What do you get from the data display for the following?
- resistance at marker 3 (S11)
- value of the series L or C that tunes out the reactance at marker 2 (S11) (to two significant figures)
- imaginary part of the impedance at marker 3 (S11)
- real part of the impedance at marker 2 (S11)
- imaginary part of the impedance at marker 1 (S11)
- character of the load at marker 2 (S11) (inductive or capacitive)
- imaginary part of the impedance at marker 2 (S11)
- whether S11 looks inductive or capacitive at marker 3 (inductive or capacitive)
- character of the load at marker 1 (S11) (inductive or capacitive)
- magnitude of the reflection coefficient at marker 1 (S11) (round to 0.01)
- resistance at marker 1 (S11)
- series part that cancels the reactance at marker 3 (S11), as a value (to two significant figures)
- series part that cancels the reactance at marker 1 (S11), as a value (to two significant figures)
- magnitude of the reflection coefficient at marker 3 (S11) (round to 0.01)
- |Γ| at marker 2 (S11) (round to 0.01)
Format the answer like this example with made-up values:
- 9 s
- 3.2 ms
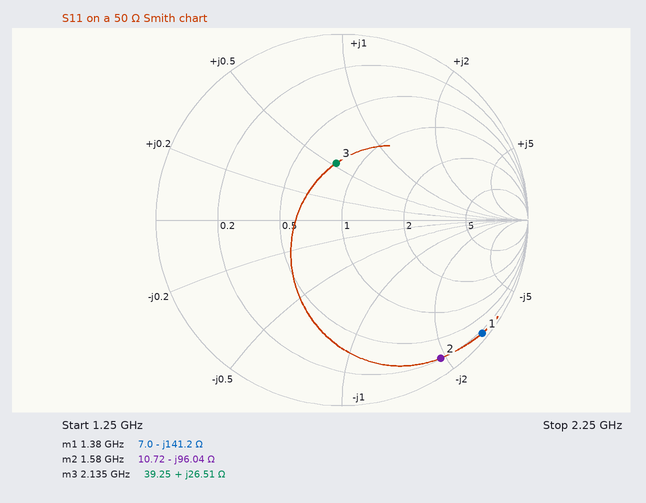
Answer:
- 39.25 Ω
- 9.7 nH
- +26.51 Ω
- 10.72 Ω
- -141.2 Ω
- capacitive
- -96.04 Ω
- inductive
- capacitive
- 0.97
- 7.0 Ω
- 2.8 pF
- 16 nH
- 0.31
- 0.91
